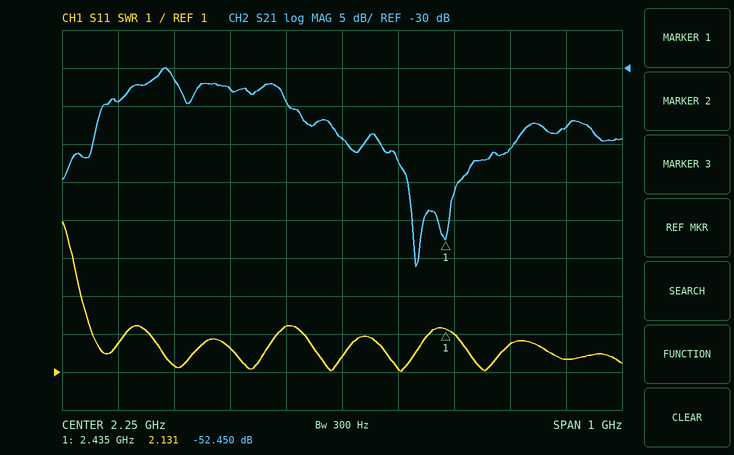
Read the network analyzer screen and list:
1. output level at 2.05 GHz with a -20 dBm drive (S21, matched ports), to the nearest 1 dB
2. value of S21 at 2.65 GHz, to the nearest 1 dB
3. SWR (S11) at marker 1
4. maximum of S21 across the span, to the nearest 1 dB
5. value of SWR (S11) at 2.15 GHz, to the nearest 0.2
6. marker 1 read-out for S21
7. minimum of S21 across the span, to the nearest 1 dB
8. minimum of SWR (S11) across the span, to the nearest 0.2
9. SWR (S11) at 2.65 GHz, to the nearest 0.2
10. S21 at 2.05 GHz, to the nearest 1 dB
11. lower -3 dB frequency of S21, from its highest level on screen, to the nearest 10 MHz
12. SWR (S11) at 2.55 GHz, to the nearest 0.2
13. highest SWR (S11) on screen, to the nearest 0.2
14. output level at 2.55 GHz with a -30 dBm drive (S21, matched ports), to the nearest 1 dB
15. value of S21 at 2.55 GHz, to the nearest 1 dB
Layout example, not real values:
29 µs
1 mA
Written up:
-53 dBm
-38 dB
2.131
-30 dB
2.2
-52.450 dB
-56 dB
1.0
1.4
-33 dB
1.87 GHz
1.8
5.0
-71 dBm
-41 dB
